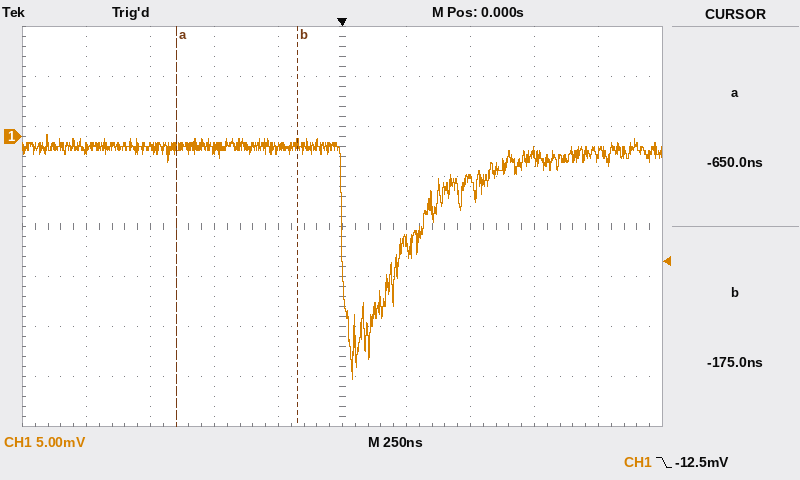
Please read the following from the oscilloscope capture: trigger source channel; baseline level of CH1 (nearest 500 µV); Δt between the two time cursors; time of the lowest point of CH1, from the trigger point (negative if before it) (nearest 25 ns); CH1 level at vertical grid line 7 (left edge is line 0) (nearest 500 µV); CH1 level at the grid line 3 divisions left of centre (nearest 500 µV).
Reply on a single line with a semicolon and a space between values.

CH1; -1.0 mV; 475 ns; +50 ns; -4.0 mV; -1.0 mV
